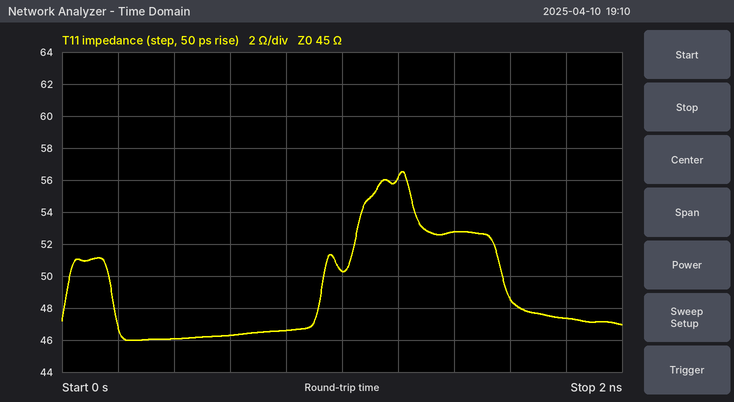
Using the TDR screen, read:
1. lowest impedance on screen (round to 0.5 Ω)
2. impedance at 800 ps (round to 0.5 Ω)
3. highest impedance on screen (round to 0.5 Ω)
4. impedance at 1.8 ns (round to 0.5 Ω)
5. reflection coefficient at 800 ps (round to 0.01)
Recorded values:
46.0 Ω
46.5 Ω
56.5 Ω
47.5 Ω
+0.02
